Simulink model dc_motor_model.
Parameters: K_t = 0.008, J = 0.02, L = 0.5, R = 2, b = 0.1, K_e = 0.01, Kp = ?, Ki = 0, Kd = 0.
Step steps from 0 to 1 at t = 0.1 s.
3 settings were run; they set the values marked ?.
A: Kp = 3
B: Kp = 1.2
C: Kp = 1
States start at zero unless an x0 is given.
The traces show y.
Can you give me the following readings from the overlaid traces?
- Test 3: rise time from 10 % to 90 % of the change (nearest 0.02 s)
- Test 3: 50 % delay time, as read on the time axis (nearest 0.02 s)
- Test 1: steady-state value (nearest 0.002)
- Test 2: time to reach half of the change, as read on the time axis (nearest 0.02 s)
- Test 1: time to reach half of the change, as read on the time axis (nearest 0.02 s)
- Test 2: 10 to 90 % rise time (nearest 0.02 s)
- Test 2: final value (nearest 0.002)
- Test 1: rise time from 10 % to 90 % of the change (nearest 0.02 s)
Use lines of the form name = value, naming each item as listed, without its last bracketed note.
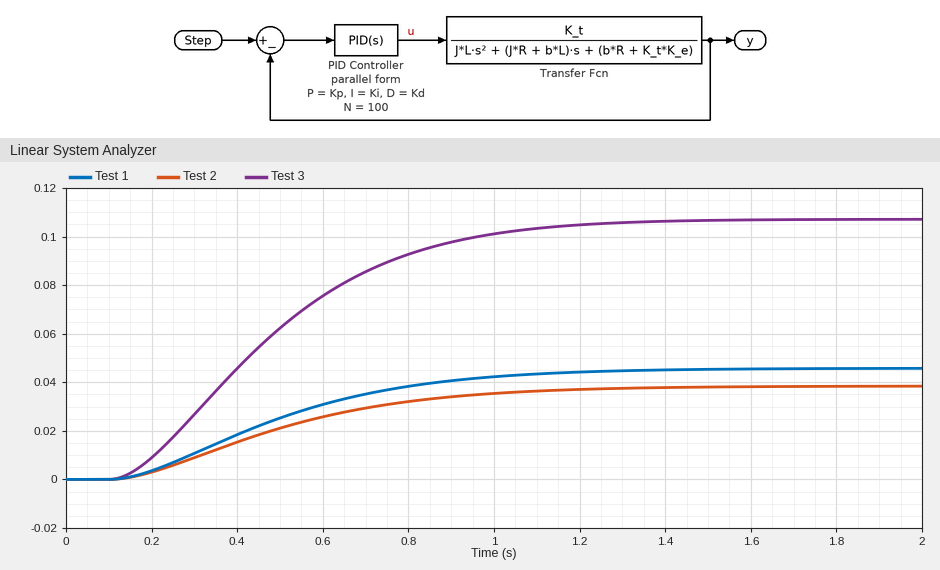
Test 3: rise time from 10 % to 90 % of the change = 0.66 s
Test 3: 50 % delay time, as read on the time axis = 0.44 s
Test 1: steady-state value = 0.046
Test 2: time to reach half of the change, as read on the time axis = 0.46 s
Test 1: time to reach half of the change, as read on the time axis = 0.46 s
Test 2: 10 to 90 % rise time = 0.72 s
Test 2: final value = 0.038
Test 1: rise time from 10 % to 90 % of the change = 0.72 s
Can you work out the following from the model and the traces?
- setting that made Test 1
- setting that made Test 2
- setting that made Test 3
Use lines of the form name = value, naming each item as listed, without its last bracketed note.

setting that made Test 1 = B
setting that made Test 2 = C
setting that made Test 3 = A
